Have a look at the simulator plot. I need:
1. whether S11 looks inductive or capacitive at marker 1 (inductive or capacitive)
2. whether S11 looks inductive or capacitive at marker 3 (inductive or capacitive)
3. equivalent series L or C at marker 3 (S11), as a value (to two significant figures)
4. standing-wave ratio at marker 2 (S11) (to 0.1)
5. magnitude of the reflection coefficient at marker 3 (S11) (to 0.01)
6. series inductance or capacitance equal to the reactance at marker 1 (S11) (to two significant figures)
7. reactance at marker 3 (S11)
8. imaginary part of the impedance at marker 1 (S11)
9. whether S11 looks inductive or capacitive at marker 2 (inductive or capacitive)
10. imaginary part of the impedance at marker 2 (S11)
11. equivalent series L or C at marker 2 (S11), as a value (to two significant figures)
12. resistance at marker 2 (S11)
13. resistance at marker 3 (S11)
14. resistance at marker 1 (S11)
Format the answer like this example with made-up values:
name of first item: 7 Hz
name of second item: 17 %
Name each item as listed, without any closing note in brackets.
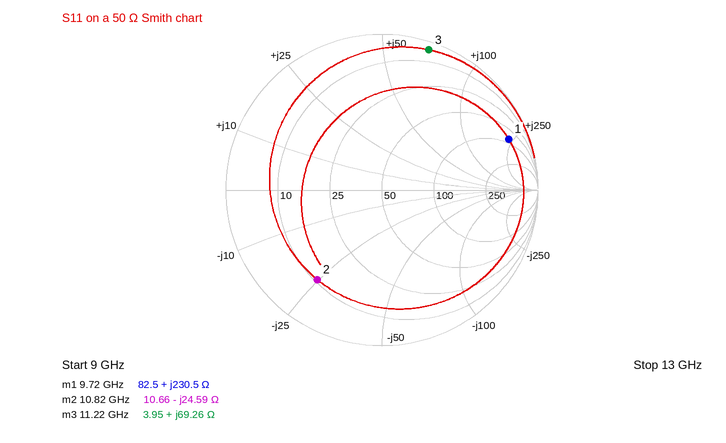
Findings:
whether S11 looks inductive or capacitive at marker 1: inductive
whether S11 looks inductive or capacitive at marker 3: inductive
equivalent series L or C at marker 3 (S11), as a value: 980 pH
standing-wave ratio at marker 2 (S11): 5.9
magnitude of the reflection coefficient at marker 3 (S11): 0.95
series inductance or capacitance equal to the reactance at marker 1 (S11): 3.8 nH
reactance at marker 3: +69.26 Ω
imaginary part of the impedance at marker 1: +230.5 Ω
whether S11 looks inductive or capacitive at marker 2: capacitive
imaginary part of the impedance at marker 2: -24.59 Ω
equivalent series L or C at marker 2 (S11), as a value: 600 fF
resistance at marker 2: 10.66 Ω
resistance at marker 3: 3.95 Ω
resistance at marker 1: 82.5 Ω
